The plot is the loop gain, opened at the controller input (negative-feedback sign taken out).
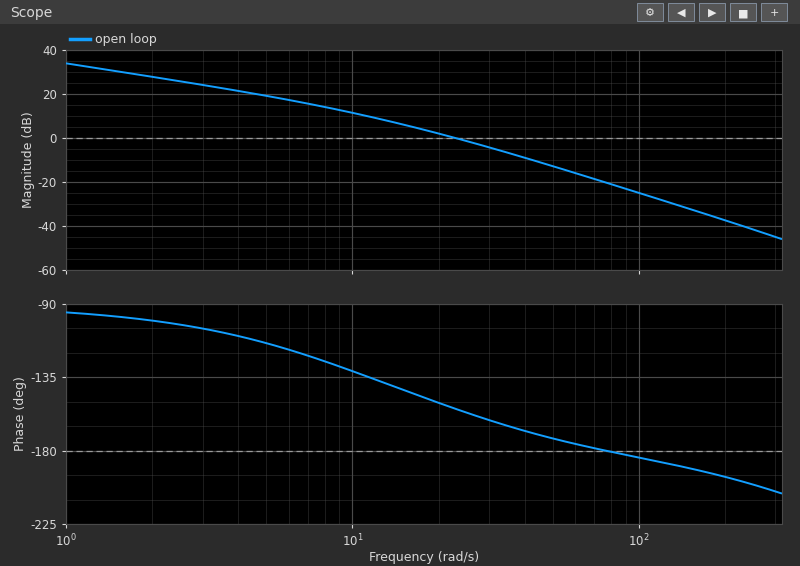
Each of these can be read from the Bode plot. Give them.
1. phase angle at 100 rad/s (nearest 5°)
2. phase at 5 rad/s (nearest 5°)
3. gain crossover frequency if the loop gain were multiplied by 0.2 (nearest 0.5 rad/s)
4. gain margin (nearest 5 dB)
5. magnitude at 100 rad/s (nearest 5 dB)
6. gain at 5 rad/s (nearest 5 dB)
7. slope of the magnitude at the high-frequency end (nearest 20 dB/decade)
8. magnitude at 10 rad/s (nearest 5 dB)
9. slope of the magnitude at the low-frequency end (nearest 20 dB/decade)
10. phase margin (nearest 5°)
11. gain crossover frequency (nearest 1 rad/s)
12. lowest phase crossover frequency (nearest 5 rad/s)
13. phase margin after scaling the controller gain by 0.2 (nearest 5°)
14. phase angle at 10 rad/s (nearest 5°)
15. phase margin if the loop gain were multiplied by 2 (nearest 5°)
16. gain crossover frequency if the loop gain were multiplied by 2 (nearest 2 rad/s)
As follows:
-185°
-115°
8.0 rad/s
20 dB
-25 dB
20 dB
-40 dB/decade
10 dB
-20 dB/decade
25°
23 rad/s
75 rad/s
55°
-130°
15°
34 rad/s
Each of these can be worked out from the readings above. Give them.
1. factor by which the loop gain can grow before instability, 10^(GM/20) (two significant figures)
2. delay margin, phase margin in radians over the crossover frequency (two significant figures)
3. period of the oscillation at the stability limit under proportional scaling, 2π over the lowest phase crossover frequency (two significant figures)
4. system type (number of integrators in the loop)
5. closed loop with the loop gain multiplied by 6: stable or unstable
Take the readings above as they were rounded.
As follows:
10
0.019 s
0.084 s
1
stable
